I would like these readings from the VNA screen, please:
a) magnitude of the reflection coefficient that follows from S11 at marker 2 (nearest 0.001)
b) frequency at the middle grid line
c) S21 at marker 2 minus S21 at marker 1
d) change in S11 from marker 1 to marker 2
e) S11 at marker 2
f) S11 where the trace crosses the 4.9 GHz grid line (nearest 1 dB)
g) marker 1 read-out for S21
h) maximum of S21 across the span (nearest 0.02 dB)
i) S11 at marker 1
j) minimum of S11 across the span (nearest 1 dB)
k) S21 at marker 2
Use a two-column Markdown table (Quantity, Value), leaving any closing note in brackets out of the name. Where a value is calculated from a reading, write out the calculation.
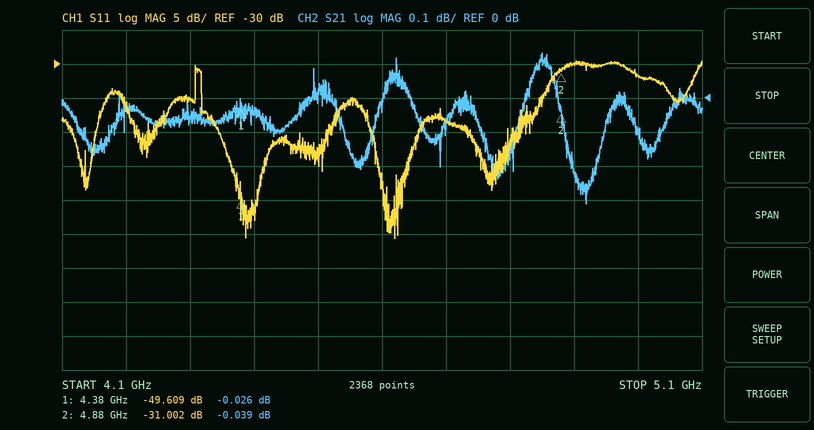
| Quantity | Value |
|---|---|
| magnitude of the reflection coefficient that follows from S11 at marker 2 | 10^(-31.002/20) ≈ 0.028 |
| frequency at the middle grid line | 4.6 GHz |
| S21 at marker 2 minus S21 at marker 1 | -0.039 − (-0.026) = -0.013 dB |
| change in S11 from marker 1 to marker 2 | -31.002 − (-49.609) = 18.607 dB |
| S11 at marker 2 | -31.002 dB |
| S11 where the trace crosses the 4.9 GHz grid line | -30 dB |
| marker 1 read-out for S21 | -0.026 dB |
| maximum of S21 across the span | 0.14 dB |
| S11 at marker 1 | -49.609 dB |
| minimum of S11 across the span | -56 dB |
| S21 at marker 2 | -0.039 dB |
